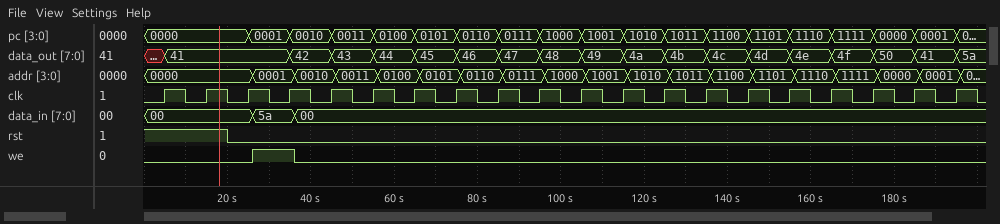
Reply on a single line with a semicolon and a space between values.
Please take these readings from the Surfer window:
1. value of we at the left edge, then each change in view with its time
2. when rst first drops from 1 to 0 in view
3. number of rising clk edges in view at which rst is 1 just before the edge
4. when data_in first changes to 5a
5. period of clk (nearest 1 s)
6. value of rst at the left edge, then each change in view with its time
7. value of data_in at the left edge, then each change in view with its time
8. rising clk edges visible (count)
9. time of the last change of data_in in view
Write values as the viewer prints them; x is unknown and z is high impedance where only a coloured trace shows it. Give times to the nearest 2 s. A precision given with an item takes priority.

0, 1 at 26 s, 0 at 36 s; 20 s; 2; 26 s; 10 s; 1, 0 at 20 s; 00, 5a at 26 s, 00 at 36 s; 20; 36 s
